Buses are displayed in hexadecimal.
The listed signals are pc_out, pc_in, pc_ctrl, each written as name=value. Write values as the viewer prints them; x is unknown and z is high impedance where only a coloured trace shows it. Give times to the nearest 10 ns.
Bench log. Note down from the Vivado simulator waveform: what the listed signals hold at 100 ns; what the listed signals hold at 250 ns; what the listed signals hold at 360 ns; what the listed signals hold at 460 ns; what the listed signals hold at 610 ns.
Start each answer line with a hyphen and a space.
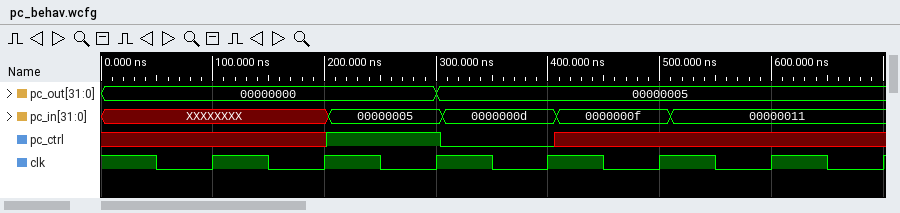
- pc_out=00000000, pc_in=XXXXXXXX, pc_ctrl=x
- pc_out=00000000, pc_in=00000005, pc_ctrl=1
- pc_out=00000005, pc_in=0000000d, pc_ctrl=0
- pc_out=00000005, pc_in=0000000f, pc_ctrl=x
- pc_out=00000005, pc_in=00000011, pc_ctrl=x
